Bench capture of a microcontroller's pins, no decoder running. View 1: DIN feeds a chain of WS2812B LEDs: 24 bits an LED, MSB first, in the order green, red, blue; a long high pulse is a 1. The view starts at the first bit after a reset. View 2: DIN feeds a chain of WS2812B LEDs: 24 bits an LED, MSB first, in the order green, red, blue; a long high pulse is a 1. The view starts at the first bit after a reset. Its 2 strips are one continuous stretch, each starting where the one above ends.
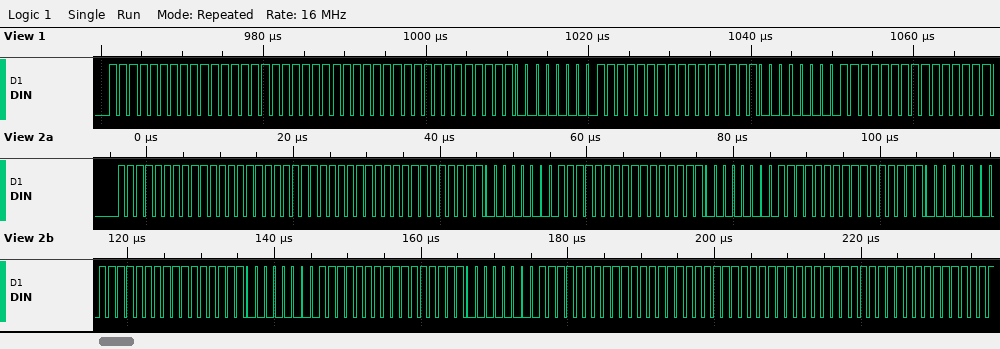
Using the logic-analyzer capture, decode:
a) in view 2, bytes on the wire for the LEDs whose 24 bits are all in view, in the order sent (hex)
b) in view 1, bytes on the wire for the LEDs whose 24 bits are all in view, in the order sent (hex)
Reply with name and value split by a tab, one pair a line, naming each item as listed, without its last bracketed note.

in view 2, bytes on the wire for the LEDs whose 24 bits are all in view, in the order sent	FF FF FF FF FF 00 FF FF 00 FF FF 00 FF FF 00 FF FF 00 FF FF FF FF FF FF
in view 1, bytes on the wire for the LEDs whose 24 bits are all in view, in the order sent	FF FF FF FF FF 00 FF FF 00
